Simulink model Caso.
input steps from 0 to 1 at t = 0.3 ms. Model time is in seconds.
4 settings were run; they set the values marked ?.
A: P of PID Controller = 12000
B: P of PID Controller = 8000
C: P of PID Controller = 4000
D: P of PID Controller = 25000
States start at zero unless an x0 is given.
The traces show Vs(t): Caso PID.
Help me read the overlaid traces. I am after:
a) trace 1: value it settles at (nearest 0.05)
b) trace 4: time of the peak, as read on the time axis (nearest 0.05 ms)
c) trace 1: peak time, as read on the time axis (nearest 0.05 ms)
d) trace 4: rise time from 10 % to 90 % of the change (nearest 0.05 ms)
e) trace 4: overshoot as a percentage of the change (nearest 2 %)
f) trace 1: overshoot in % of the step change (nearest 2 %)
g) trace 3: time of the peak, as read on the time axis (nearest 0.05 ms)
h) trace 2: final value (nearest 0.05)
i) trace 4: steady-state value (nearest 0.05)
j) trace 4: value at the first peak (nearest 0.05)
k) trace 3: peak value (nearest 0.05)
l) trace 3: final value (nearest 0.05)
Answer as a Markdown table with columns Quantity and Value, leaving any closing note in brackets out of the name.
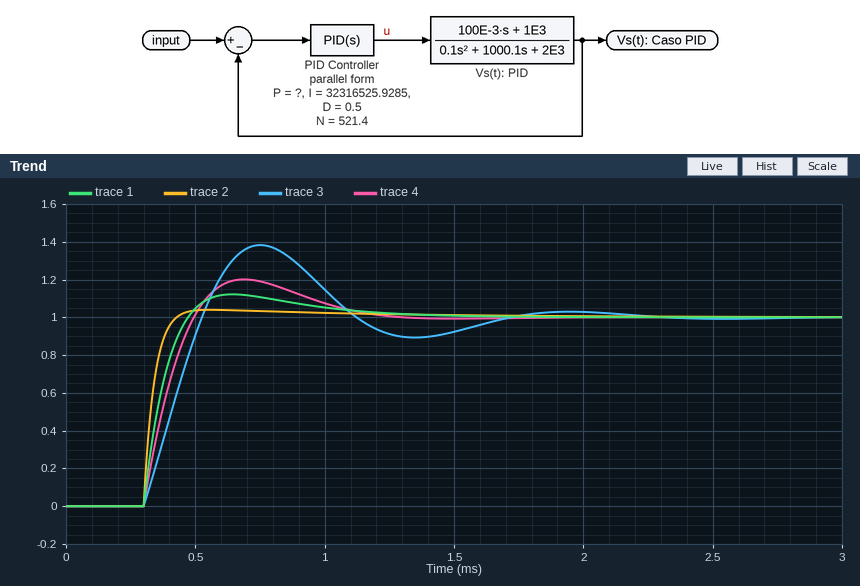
| Quantity | Value |
|---|---|
| trace 1: value it settles at | 1.00 |
| trace 4: time of the peak, as read on the time axis | 0.70 ms |
| trace 1: peak time, as read on the time axis | 0.65 ms |
| trace 4: rise time from 10 % to 90 % of the change | 0.15 ms |
| trace 4: overshoot as a percentage of the change | 20 % |
| trace 1: overshoot in % of the step change | 12 % |
| trace 3: time of the peak, as read on the time axis | 0.75 ms |
| trace 2: final value | 1.00 |
| trace 4: steady-state value | 1.00 |
| trace 4: value at the first peak | 1.20 |
| trace 3: peak value | 1.40 |
| trace 3: final value | 1.00 |
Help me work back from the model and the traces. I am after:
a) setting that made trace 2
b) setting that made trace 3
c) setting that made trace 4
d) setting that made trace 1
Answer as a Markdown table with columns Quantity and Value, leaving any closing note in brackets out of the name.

| Quantity | Value |
|---|---|
| setting that made trace 2 | D |
| setting that made trace 3 | C |
| setting that made trace 4 | B |
| setting that made trace 1 | A |
